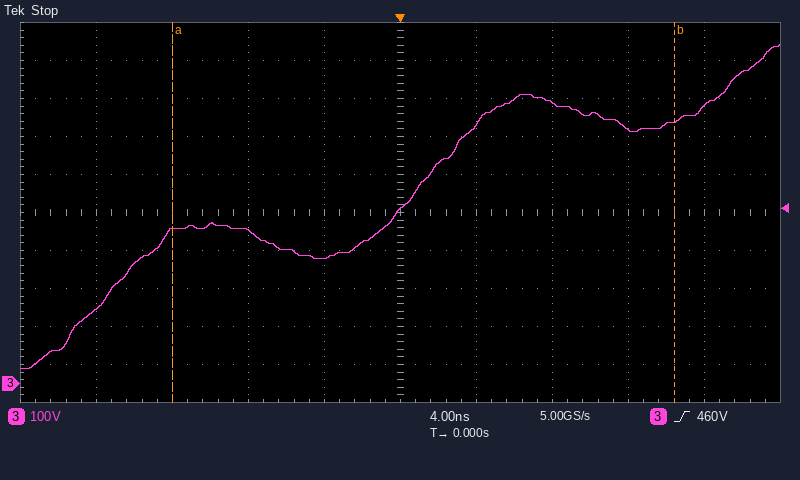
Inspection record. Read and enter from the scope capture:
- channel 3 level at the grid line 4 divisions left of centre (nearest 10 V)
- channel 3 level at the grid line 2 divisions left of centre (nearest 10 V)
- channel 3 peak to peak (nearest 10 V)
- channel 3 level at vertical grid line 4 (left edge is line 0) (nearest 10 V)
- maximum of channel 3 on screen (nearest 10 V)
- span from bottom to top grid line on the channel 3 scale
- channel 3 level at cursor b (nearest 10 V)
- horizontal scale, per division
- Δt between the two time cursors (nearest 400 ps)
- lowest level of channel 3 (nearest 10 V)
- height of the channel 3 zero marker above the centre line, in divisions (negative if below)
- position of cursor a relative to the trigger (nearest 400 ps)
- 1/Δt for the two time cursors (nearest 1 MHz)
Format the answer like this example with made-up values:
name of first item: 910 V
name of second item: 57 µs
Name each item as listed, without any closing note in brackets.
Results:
channel 3 level at the grid line 4 divisions left of centre: 200 V
channel 3 level at the grid line 2 divisions left of centre: 400 V
channel 3 peak to peak: 850 V
channel 3 level at vertical grid line 4 (left edge is line 0): 330 V
maximum of channel 3 on screen: 890 V
span from bottom to top grid line on the channel 3 scale: 1 kV
channel 3 level at cursor b: 690 V
horizontal scale, per division: 4 ns
Δt between the two time cursors: 26.4 ns
lowest level of channel 3: 40 V
height of the channel 3 zero marker above the centre line, in divisions: -4.5 div
position of cursor a relative to the trigger: -12.0 ns
1/Δt for the two time cursors: 38 MHz
